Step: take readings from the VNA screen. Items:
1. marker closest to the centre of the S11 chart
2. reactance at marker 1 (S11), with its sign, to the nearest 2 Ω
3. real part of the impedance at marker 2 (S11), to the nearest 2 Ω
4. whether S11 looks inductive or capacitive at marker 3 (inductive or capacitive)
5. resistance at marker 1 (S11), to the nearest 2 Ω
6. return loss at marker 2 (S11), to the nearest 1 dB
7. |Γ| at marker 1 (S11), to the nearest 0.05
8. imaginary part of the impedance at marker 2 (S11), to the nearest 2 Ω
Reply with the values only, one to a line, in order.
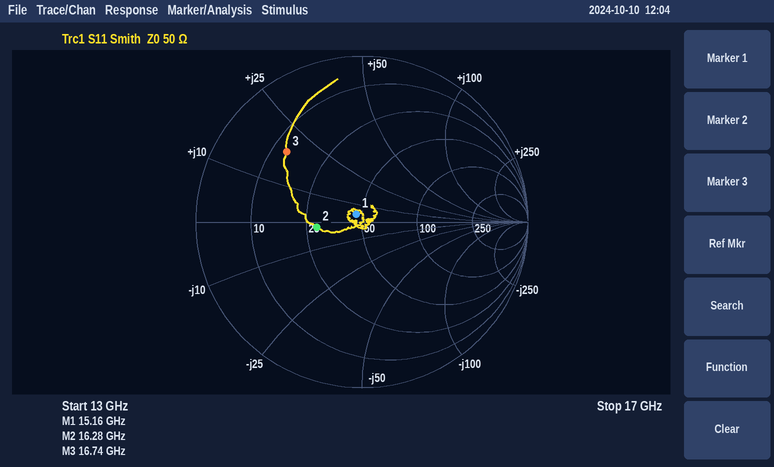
marker 1
+4 Ω
28 Ω
inductive
46 Ω
11 dB
0.05
-2 Ω
